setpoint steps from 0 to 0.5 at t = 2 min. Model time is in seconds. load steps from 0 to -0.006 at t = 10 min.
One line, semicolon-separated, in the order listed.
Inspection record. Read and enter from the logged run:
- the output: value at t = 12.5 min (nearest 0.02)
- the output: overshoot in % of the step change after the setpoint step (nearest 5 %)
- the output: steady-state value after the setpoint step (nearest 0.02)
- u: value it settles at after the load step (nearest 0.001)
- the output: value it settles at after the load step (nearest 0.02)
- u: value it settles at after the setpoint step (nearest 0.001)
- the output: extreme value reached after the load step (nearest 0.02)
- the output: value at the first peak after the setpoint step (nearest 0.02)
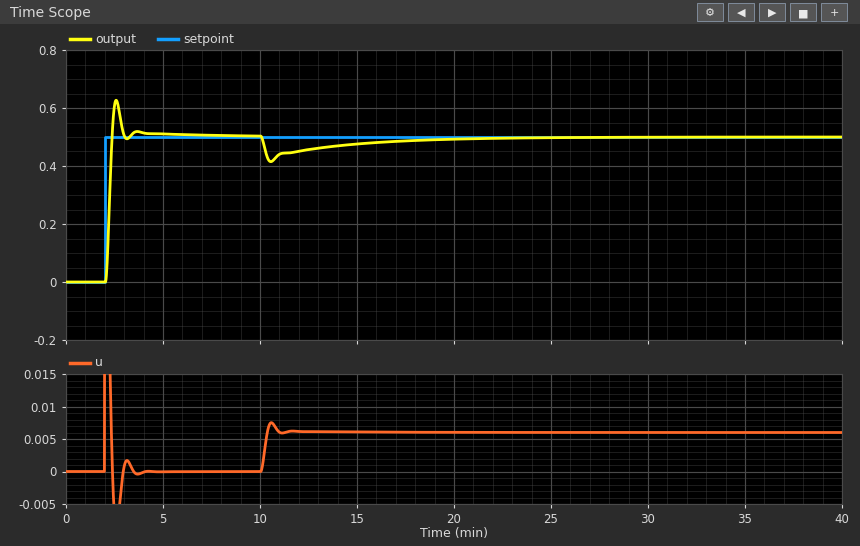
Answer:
0.46; 25 %; 0.50; 0.006; 0.50; 0.000; 0.42; 0.62
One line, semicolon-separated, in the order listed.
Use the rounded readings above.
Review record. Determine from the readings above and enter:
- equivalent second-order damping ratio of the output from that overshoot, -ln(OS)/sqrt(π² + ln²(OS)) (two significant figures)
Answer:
0.40
